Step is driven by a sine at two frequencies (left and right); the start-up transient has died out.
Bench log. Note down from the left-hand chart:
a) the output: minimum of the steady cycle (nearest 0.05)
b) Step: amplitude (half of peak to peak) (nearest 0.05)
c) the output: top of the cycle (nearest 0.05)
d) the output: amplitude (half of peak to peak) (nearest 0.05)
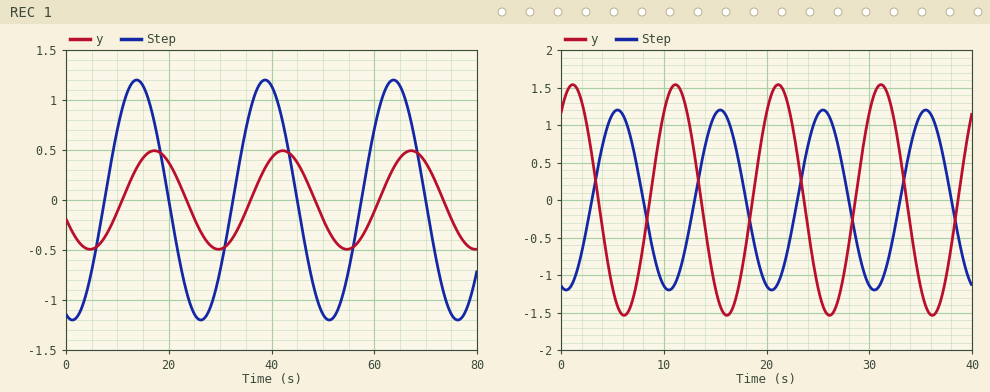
-0.50
1.20
0.50
0.50
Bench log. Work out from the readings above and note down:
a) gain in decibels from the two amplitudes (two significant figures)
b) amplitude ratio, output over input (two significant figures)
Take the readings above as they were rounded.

-7.6 dB
0.42
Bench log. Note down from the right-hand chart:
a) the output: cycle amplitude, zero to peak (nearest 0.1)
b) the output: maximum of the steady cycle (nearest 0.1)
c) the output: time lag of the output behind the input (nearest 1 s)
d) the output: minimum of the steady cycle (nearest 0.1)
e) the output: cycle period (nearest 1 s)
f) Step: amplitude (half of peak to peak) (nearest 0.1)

1.5
1.5
6 s
-1.5
10 s
1.2
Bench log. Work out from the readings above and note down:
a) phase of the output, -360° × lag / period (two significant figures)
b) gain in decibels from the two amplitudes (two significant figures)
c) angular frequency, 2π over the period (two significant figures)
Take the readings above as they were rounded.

-220°
1.9 dB
0.63 rad/s
